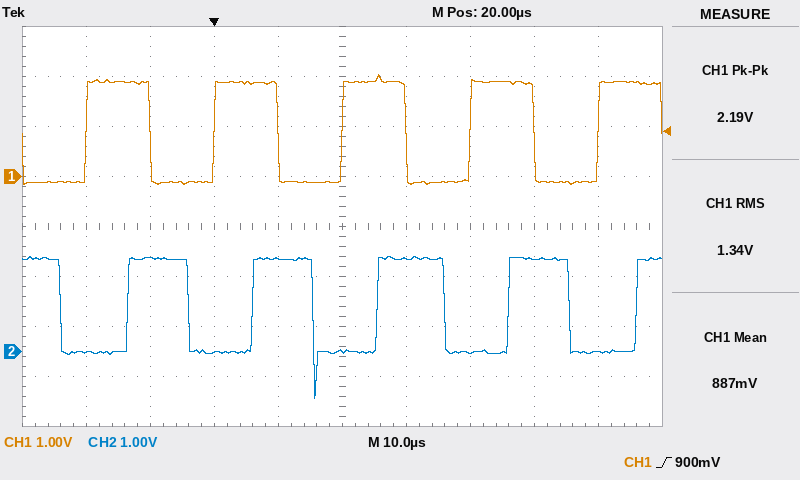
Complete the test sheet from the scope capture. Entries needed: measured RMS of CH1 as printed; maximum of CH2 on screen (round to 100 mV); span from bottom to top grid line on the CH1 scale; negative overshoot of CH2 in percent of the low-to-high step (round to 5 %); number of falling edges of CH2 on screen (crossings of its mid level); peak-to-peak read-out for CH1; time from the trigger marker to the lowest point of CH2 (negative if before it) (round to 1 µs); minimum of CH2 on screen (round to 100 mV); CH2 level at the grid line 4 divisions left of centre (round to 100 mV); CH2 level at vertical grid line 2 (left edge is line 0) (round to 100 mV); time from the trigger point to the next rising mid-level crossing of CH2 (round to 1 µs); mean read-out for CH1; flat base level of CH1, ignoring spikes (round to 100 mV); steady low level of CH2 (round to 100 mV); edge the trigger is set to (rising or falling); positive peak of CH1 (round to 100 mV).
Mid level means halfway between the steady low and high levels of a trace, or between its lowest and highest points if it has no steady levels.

1.34 V
1.9 V
8 V
50 %
5
2.19 V
+16 µs
-900 mV
0.0 V
1.9 V
6 µs
887 mV
-100 mV
0.0 V
rising
2.0 V
